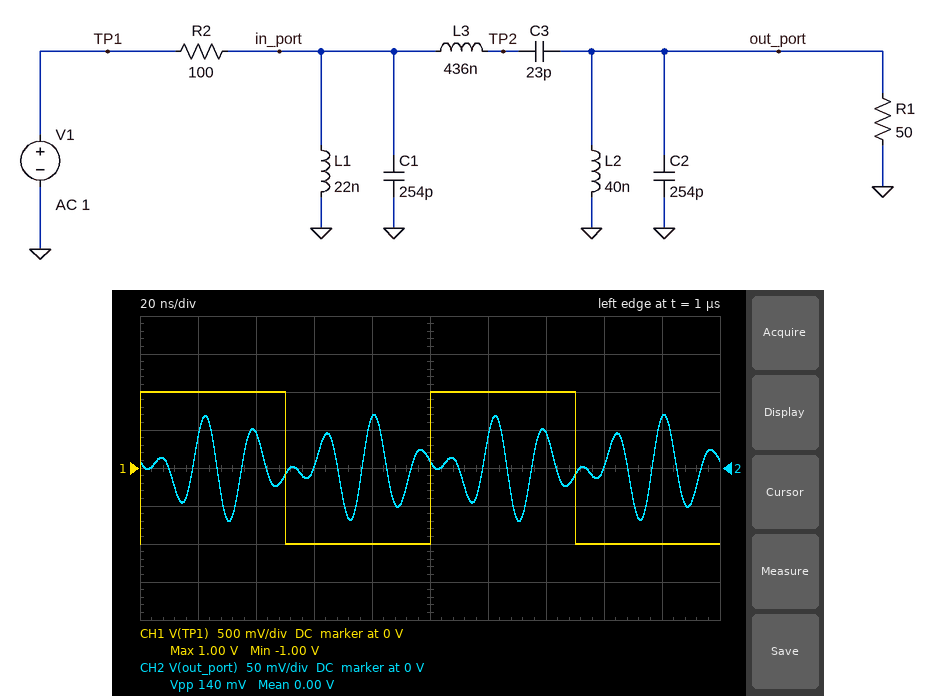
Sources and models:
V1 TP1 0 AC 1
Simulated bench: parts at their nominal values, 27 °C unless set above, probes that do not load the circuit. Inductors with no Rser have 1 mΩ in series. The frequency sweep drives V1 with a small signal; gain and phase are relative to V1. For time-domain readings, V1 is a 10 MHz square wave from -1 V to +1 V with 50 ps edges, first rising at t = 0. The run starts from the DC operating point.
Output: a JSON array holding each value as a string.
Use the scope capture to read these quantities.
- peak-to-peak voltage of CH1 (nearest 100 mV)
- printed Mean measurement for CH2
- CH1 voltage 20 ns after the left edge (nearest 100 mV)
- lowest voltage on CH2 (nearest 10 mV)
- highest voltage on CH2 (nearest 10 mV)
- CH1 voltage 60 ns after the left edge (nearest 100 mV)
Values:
["2.0 V", "0.00 V", "1.0 V", "-70 mV", "70 mV", "-1.0 V"]
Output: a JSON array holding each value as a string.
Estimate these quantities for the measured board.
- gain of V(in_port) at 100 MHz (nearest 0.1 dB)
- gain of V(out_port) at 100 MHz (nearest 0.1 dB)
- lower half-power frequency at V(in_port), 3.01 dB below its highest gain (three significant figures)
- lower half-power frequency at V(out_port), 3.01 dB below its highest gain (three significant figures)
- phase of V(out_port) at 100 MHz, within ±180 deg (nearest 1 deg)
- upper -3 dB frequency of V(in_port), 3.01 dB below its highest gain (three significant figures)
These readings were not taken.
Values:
["-18.4 dB", "-45.9 dB", "68.6 MHz", "50.5 MHz", "107 deg", "74.4 MHz"]
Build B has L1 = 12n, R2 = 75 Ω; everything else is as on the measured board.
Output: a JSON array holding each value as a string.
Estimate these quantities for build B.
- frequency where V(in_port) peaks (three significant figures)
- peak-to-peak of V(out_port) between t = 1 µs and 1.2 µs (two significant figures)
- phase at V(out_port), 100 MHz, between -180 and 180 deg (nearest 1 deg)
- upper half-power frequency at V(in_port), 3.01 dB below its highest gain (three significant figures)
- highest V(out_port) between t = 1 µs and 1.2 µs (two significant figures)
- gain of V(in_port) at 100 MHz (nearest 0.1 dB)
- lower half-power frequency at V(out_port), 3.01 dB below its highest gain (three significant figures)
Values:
["93.0 MHz", "56 mV", "131 deg", "97.2 MHz", "28 mV", "-5.7 dB", "51.6 MHz"]
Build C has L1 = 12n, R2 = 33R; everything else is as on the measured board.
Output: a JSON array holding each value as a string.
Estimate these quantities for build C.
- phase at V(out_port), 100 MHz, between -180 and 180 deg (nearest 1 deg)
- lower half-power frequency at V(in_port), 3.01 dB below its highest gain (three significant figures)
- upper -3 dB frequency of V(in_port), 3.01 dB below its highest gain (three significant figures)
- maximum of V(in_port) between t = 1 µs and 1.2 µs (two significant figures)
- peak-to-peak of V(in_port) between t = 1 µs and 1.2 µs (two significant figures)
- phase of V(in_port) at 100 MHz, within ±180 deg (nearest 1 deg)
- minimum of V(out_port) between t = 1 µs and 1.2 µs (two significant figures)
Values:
["154 deg", "84.2 MHz", "103 MHz", "370 mV", "740 mV", "-36 deg", "-58 mV"]
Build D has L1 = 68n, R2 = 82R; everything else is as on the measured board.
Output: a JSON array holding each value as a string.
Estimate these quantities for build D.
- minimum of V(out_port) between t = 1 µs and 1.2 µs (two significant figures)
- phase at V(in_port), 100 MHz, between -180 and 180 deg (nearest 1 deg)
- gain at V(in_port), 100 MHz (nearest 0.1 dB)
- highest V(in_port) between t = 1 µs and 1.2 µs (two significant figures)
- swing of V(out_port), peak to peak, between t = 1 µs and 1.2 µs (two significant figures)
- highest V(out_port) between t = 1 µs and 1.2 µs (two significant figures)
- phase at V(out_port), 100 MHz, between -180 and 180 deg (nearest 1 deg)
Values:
["-85 mV", "-85 deg", "-20.7 dB", "340 mV", "170 mV", "85 mV", "105 deg"]
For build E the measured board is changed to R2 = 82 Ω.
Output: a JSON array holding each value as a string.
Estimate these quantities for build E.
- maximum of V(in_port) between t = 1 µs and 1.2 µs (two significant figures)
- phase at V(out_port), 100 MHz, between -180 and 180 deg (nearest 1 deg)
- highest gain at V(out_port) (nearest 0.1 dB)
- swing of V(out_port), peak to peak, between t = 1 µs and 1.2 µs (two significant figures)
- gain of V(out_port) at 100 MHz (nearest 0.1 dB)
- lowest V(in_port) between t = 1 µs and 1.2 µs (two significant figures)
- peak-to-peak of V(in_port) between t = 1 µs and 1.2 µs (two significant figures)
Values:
["280 mV", "108 deg", "-12.2 dB", "160 mV", "-44.2 dB", "-280 mV", "560 mV"]
